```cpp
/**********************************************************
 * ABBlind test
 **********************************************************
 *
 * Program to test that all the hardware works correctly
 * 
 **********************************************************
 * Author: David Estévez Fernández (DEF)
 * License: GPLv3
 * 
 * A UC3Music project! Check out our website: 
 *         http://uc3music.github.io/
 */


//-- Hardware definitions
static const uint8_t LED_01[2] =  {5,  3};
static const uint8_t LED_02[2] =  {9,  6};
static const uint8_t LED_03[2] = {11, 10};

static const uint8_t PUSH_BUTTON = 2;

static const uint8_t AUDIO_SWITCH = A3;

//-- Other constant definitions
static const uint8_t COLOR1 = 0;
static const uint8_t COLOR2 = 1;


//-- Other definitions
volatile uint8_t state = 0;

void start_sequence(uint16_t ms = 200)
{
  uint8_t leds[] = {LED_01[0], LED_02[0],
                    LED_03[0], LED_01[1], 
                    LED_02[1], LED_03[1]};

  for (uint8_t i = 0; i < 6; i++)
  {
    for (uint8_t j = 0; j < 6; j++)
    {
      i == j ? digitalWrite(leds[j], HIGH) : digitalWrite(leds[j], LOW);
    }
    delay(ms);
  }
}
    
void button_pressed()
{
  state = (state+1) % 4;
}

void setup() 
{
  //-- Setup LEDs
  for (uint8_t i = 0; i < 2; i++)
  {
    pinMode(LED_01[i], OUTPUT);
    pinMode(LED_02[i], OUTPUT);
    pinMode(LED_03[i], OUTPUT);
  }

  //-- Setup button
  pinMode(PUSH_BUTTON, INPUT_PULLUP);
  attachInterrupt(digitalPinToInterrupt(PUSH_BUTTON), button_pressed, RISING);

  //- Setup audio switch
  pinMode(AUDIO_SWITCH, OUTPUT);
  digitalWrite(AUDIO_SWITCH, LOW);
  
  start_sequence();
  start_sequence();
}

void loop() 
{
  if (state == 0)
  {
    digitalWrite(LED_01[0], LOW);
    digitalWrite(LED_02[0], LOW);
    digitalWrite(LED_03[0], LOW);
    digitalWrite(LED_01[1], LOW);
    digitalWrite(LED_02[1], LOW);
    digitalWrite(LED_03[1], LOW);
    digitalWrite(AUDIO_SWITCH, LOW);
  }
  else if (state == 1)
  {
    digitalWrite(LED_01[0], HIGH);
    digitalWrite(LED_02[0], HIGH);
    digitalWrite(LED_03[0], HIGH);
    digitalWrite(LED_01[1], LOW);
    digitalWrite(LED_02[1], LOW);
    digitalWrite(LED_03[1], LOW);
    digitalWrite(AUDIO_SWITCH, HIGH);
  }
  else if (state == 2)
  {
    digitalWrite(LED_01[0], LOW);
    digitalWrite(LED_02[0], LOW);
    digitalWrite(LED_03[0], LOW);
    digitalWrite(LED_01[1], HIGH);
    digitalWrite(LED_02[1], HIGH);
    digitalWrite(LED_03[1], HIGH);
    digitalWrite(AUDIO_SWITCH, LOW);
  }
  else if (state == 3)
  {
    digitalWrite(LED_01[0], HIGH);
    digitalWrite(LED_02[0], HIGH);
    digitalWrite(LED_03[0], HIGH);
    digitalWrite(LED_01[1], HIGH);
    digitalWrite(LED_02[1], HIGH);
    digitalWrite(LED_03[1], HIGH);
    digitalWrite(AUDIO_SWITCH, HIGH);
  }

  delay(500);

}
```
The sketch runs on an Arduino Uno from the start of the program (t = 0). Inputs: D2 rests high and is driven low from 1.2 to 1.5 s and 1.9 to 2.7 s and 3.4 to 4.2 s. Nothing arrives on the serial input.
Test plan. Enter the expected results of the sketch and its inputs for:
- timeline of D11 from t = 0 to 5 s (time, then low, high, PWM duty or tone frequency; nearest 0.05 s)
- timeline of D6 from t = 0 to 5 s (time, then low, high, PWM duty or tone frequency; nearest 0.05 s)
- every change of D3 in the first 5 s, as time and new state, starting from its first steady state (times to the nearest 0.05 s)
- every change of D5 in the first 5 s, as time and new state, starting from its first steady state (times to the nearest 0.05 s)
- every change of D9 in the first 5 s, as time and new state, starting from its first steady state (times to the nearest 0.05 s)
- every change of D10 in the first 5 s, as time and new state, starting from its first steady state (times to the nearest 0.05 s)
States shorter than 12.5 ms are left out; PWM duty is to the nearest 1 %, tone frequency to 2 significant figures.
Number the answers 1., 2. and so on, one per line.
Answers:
1. 0 s low; 0.4 s high; 0.6 s low; 1.6 s high; 1.8 s low; 2.4 s high; 2.9 s low; 4.4 s high
2. 0 s low; 0.8 s high; 1 s low; 2 s high; 2.2 s low; 2.9 s high
3. 0 s low; 0.6 s high; 0.8 s low; 1.8 s high; 2 s low; 2.9 s high
4. 0 s high; 0.2 s low; 1.2 s high; 1.4 s low; 2.4 s high; 2.9 s low; 4.4 s high
5. 0 s low; 0.2 s high; 0.4 s low; 1.4 s high; 1.6 s low; 2.4 s high; 2.9 s low; 4.4 s high
6. 0 s low; 1 s high; 1.2 s low; 2.2 s high; 2.4 s low; 2.9 s high
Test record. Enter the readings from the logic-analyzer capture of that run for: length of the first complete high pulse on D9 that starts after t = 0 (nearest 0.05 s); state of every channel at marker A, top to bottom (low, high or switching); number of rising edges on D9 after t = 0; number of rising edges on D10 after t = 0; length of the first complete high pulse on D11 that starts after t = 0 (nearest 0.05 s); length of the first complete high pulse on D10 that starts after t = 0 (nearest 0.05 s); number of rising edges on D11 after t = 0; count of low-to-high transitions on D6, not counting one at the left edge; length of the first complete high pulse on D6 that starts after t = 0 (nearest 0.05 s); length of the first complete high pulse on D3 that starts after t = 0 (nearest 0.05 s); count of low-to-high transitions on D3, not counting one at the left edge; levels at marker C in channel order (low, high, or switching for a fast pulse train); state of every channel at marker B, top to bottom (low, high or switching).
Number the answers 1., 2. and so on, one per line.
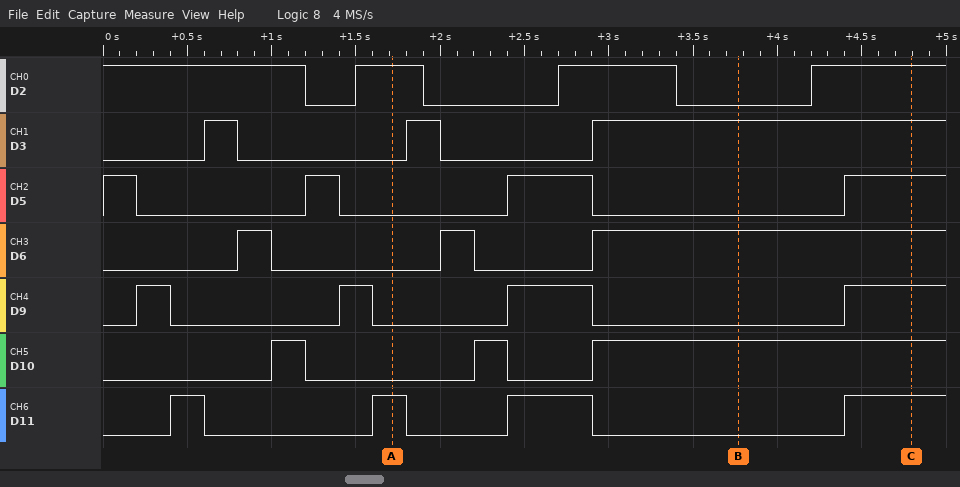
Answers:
1. 0.20 s
2. D2 high, D3 low, D5 low, D6 low, D9 low, D10 low, D11 high
3. 4
4. 3
5. 0.20 s
6. 0.20 s
7. 4
8. 3
9. 0.20 s
10. 0.20 s
11. 3
12. D2 high, D3 high, D5 high, D6 high, D9 high, D10 high, D11 high
13. D2 low, D3 high, D5 low, D6 high, D9 low, D10 high, D11 low
